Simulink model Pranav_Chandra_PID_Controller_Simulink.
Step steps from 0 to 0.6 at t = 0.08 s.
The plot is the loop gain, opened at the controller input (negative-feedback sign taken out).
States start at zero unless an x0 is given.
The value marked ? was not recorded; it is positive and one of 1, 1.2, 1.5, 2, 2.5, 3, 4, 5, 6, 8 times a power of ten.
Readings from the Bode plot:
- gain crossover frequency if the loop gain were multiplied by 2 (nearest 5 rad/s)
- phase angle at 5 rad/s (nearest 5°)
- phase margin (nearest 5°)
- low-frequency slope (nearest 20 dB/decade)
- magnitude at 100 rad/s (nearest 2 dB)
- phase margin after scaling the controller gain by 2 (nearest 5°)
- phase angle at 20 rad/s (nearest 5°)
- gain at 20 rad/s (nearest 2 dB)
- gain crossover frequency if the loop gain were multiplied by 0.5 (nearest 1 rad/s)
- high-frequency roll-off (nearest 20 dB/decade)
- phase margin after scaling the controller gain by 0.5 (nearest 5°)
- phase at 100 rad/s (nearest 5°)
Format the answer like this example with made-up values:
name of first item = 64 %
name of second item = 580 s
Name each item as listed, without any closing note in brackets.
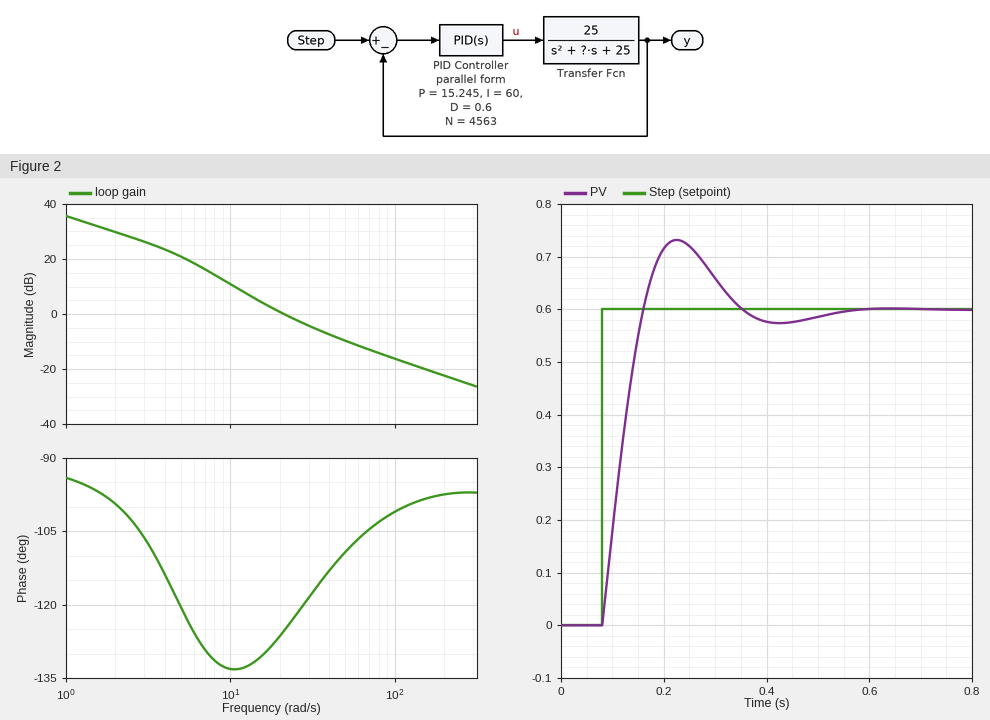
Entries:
gain crossover frequency if the loop gain were multiplied by 2 = 35 rad/s
phase angle at 5 rad/s = -120°
phase margin = 55°
low-frequency slope = -20 dB/decade
magnitude at 100 rad/s = -16 dB
phase margin after scaling the controller gain by 2 = 65°
phase angle at 20 rad/s = -125°
gain at 20 rad/s = 0 dB
gain crossover frequency if the loop gain were multiplied by 0.5 = 14 rad/s
high-frequency roll-off = -20 dB/decade
phase margin after scaling the controller gain by 0.5 = 50°
phase at 100 rad/s = -100°
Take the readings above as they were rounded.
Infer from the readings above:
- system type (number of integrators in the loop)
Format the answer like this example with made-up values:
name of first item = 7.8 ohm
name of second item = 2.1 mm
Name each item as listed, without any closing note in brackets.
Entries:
system type = 1
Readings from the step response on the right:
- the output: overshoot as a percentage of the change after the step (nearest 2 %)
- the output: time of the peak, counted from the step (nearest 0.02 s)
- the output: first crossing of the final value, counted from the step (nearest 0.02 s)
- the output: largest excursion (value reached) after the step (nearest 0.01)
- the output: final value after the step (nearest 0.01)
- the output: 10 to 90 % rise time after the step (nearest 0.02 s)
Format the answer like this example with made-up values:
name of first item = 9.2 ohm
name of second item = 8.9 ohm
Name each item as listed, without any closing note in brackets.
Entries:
the output: overshoot as a percentage of the change after the step = 22 %
the output: time of the peak, counted from the step = 0.14 s
the output: first crossing of the final value, counted from the step = 0.08 s
the output: largest excursion (value reached) after the step = 0.73
the output: final value after the step = 0.60
the output: 10 to 90 % rise time after the step = 0.06 s
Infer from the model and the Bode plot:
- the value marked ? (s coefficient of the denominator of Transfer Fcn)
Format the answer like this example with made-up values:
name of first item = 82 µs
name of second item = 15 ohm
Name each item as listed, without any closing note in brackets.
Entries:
the value marked ? = 8
